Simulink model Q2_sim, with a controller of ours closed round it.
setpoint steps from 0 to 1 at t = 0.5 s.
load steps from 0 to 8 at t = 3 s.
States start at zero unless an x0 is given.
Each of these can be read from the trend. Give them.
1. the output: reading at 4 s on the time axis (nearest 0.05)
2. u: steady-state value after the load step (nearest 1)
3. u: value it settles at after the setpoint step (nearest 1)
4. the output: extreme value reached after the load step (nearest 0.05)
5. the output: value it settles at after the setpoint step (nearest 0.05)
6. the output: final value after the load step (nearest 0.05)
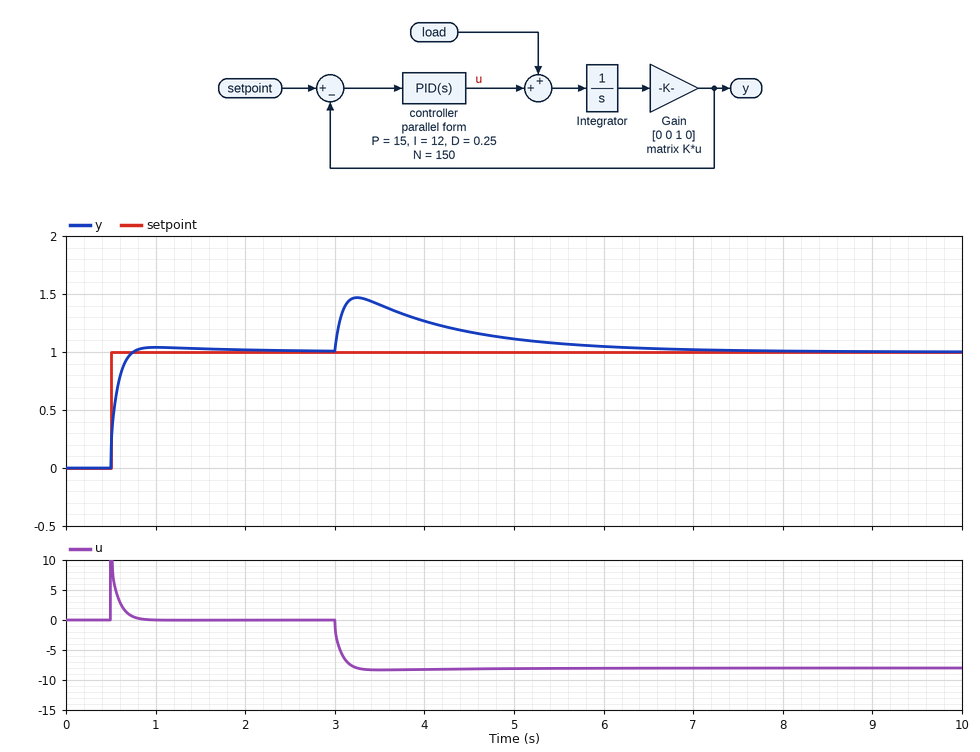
1.25
-8
0
1.45
1.00
1.00
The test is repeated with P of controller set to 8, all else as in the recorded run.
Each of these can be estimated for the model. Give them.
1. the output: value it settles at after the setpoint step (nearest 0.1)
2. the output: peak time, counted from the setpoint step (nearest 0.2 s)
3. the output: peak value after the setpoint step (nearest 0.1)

1.0
0.6 s
1.1
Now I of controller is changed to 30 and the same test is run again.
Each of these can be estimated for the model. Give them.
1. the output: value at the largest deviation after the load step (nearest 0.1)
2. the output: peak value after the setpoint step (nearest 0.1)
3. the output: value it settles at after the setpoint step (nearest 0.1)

1.4
1.1
1.0
